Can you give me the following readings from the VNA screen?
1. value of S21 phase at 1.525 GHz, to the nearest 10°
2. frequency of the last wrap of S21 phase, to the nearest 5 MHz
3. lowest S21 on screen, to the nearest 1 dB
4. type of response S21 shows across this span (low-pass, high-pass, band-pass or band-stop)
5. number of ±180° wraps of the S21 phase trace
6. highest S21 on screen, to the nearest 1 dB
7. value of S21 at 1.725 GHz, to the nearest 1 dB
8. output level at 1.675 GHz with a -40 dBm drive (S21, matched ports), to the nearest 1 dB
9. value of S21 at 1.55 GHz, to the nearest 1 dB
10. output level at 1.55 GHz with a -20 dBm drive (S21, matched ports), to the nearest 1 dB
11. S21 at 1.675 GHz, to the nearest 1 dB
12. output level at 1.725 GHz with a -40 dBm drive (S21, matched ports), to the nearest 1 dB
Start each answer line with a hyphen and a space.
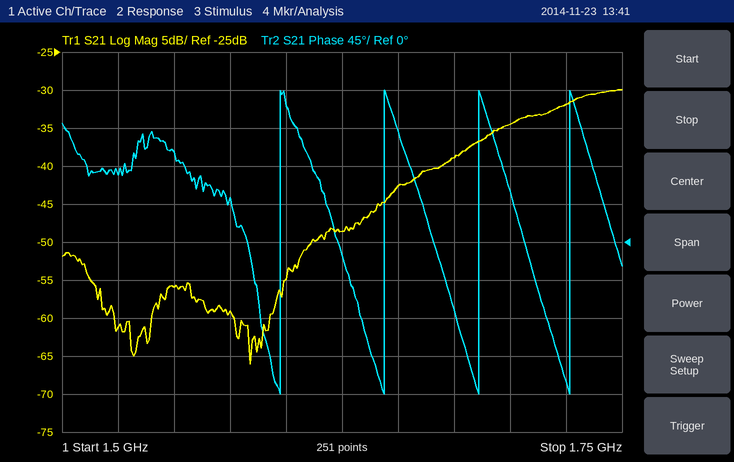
- 80°
- 1.725 GHz
- -66 dB
- high-pass
- 4
- -30 dB
- -32 dB
- -79 dBm
- -56 dB
- -76 dBm
- -39 dB
- -72 dBm
